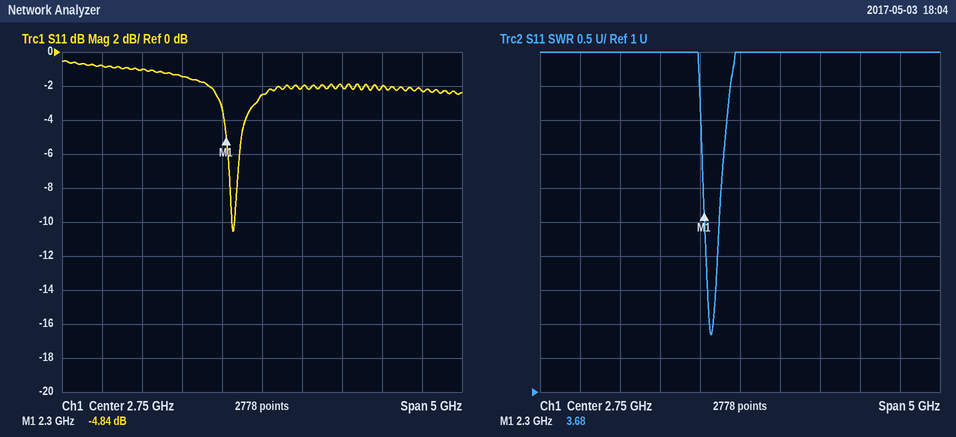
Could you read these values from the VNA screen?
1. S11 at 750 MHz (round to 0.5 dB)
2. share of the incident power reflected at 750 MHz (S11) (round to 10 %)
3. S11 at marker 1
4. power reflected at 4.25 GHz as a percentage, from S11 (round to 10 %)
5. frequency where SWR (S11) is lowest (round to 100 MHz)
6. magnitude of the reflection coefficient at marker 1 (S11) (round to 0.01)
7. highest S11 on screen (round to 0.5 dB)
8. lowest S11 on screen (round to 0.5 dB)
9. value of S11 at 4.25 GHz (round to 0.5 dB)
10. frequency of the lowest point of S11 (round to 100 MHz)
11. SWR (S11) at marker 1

-1.0 dB
80 %
-4.84 dB
60 %
2.4 GHz
0.57
-0.5 dB
-10.5 dB
-2.0 dB
2.4 GHz
3.68
